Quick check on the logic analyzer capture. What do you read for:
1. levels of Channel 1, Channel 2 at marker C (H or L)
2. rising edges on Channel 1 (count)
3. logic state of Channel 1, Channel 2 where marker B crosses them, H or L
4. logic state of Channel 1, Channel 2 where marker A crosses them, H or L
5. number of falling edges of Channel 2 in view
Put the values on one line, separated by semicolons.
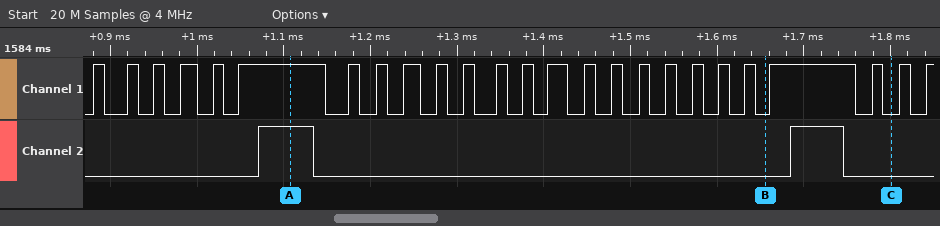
Channel 1=L, Channel 2=L; 25; Channel 1=L, Channel 2=L; Channel 1=H, Channel 2=H; 2
